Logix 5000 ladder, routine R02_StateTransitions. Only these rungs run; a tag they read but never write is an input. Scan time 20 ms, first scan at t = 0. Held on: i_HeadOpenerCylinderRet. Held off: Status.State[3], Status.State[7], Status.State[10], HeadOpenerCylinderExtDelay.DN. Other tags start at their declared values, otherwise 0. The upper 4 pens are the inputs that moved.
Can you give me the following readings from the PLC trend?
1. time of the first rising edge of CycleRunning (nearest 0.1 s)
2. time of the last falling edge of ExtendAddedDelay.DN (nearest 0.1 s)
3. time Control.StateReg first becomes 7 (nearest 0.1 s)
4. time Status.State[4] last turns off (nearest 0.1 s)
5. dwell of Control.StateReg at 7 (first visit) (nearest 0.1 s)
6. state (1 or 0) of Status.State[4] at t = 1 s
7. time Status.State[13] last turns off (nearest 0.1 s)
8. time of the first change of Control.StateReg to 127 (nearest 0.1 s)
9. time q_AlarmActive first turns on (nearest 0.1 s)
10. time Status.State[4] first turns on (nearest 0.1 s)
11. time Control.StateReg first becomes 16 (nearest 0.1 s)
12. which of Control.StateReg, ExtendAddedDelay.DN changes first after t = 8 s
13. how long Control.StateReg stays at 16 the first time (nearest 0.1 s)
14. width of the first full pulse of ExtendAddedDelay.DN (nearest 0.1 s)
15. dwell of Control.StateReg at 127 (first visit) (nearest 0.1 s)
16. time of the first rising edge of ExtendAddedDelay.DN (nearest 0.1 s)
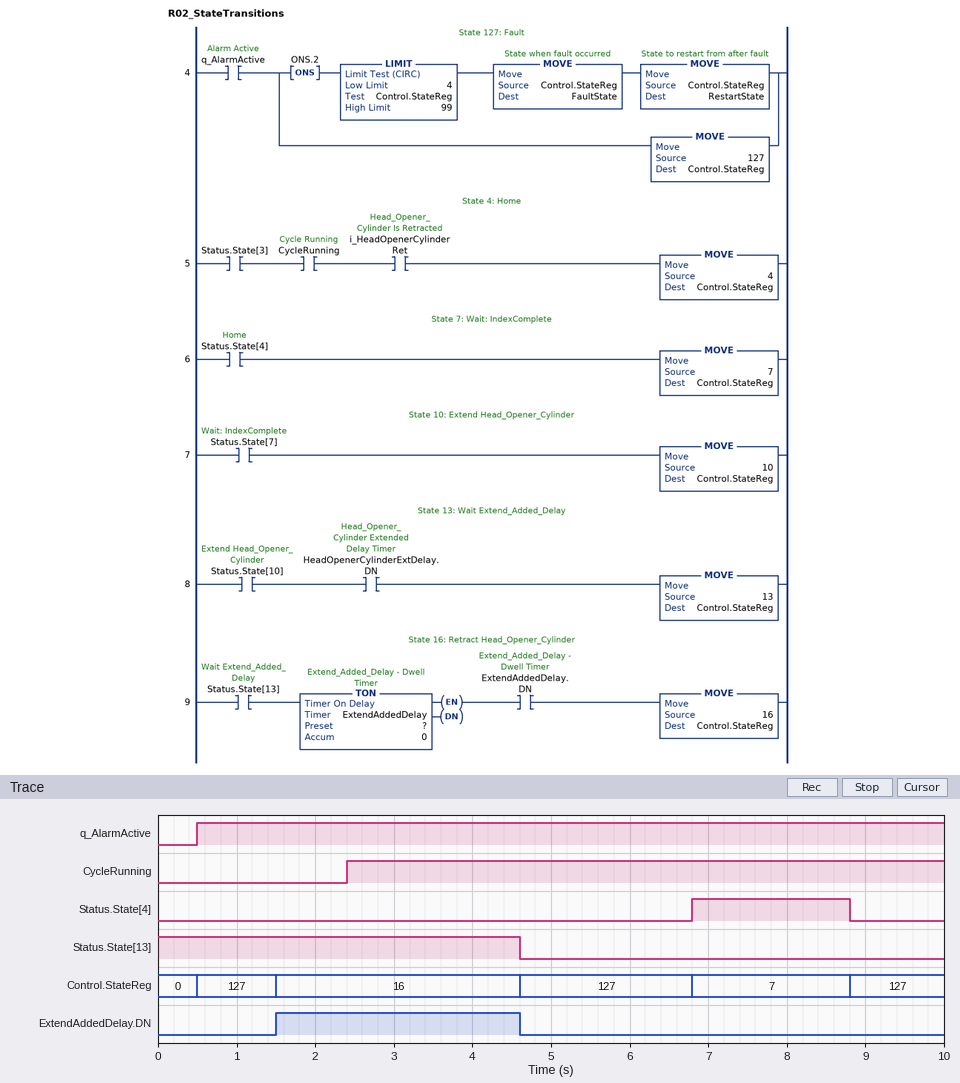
2.4 s
4.6 s
6.8 s
8.8 s
2.0 s
0
4.6 s
0.5 s
0.5 s
6.8 s
1.5 s
Control.StateReg
3.1 s
3.1 s
1.0 s
1.5 s
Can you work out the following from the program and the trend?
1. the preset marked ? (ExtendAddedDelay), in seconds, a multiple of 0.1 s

1.5 s
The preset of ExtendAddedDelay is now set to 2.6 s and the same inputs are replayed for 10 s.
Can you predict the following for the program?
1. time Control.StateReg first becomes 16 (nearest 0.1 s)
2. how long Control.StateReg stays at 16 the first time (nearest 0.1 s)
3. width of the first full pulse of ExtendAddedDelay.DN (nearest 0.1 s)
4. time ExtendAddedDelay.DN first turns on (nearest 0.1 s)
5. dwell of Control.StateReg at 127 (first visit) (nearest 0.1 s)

2.6 s
2.0 s
2.0 s
2.6 s
2.1 s
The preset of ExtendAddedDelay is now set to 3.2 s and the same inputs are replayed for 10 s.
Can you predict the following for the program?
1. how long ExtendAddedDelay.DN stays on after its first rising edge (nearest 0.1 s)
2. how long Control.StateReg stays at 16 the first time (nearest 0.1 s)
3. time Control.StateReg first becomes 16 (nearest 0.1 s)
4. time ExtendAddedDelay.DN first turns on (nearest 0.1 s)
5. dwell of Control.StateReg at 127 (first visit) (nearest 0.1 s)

1.4 s
1.4 s
3.2 s
3.2 s
2.7 s
